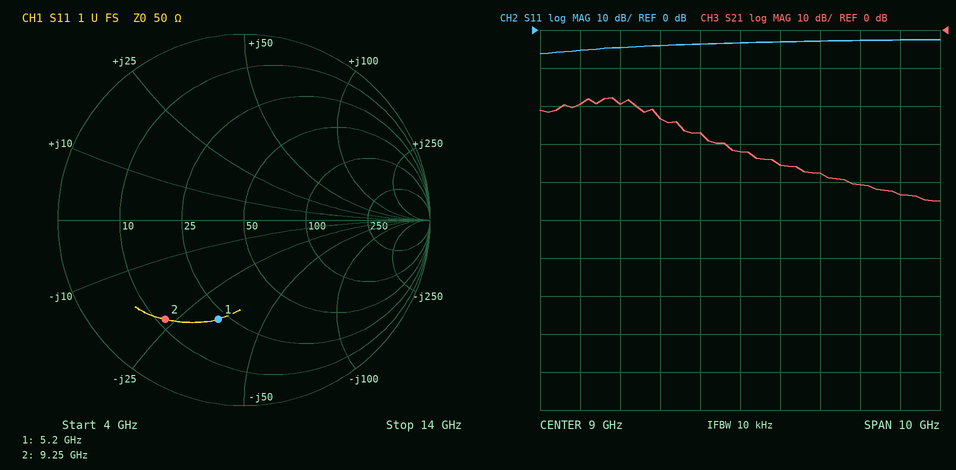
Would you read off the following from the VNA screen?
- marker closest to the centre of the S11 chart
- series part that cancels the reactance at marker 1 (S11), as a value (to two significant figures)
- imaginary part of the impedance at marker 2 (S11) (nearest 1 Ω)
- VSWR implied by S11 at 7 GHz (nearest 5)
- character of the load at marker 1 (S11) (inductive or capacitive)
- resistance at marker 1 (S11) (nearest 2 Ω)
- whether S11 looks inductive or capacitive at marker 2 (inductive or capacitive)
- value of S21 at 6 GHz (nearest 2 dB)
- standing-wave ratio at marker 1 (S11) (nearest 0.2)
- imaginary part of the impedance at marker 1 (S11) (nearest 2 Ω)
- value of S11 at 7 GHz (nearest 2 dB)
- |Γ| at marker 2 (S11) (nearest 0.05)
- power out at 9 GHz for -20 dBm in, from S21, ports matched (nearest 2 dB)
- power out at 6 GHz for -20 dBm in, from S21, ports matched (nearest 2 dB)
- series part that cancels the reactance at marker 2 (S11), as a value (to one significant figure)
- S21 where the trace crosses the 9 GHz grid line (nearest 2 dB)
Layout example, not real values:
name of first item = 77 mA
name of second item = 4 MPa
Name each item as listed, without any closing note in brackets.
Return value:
marker closest to the centre of the S11 chart = marker 1
series part that cancels the reactance at marker 1 (S11), as a value = 1.0 nH
imaginary part of the impedance at marker 2 (S11) = -23 Ω
VSWR implied by S11 at 7 GHz = 5
character of the load at marker 1 (S11) = capacitive
resistance at marker 1 (S11) = 22 Ω
whether S11 looks inductive or capacitive at marker 2 = capacitive
value of S21 at 6 GHz = -20 dB
standing-wave ratio at marker 1 (S11) = 3.4
imaginary part of the impedance at marker 1 (S11) = -34 Ω
value of S11 at 7 GHz = -4 dB
|Γ| at marker 2 (S11) = 0.70
power out at 9 GHz for -20 dBm in, from S21, ports matched = -52 dBm
power out at 6 GHz for -20 dBm in, from S21, ports matched = -40 dBm
series part that cancels the reactance at marker 2 (S11), as a value = 400 pH
S21 where the trace crosses the 9 GHz grid line = -32 dB
